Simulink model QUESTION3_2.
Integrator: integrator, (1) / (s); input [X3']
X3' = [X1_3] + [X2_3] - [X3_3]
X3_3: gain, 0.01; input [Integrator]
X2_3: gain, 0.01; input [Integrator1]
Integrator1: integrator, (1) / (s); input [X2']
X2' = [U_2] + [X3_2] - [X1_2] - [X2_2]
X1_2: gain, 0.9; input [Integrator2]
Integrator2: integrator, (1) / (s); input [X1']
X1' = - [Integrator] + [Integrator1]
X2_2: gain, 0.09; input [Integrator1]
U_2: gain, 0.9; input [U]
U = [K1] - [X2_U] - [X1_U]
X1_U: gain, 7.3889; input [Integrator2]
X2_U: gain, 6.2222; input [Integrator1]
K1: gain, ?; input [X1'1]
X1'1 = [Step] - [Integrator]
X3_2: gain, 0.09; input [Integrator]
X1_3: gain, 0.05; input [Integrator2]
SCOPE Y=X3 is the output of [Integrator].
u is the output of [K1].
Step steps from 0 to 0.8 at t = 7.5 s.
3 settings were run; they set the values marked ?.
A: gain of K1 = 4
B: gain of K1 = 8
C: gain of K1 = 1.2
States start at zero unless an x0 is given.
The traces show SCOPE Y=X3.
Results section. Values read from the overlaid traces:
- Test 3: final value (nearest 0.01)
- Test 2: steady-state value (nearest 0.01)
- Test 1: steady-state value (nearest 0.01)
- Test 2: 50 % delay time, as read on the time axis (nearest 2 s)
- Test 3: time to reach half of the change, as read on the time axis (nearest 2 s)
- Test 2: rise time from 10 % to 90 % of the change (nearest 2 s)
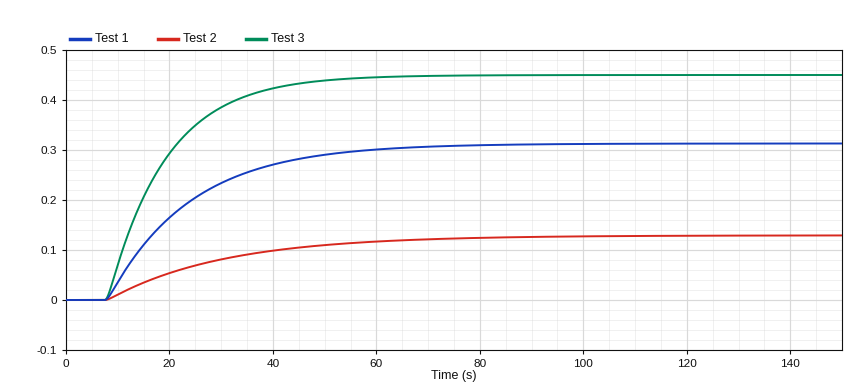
0.45
0.13
0.31
24 s
16 s
48 s
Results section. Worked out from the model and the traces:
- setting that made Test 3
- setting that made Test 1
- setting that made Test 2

B
A
C
